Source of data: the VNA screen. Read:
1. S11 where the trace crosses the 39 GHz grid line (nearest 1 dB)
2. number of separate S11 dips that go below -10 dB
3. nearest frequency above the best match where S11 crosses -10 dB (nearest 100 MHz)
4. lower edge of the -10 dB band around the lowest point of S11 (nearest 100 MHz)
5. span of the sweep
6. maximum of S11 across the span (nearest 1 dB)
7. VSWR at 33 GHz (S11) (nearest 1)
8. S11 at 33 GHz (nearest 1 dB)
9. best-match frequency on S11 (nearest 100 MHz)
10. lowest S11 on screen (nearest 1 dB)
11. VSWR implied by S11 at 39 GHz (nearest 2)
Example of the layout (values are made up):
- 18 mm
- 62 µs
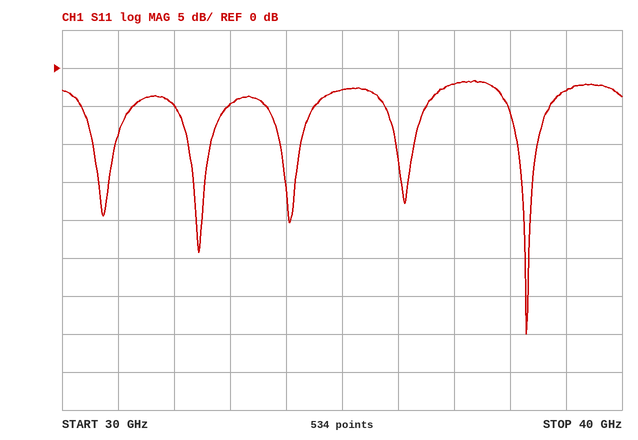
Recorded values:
- -3 dB
- 5
- 38.5 GHz
- 38.1 GHz
- 10 GHz
- -2 dB
- 4
- -5 dB
- 38.3 GHz
- -35 dB
- 6
